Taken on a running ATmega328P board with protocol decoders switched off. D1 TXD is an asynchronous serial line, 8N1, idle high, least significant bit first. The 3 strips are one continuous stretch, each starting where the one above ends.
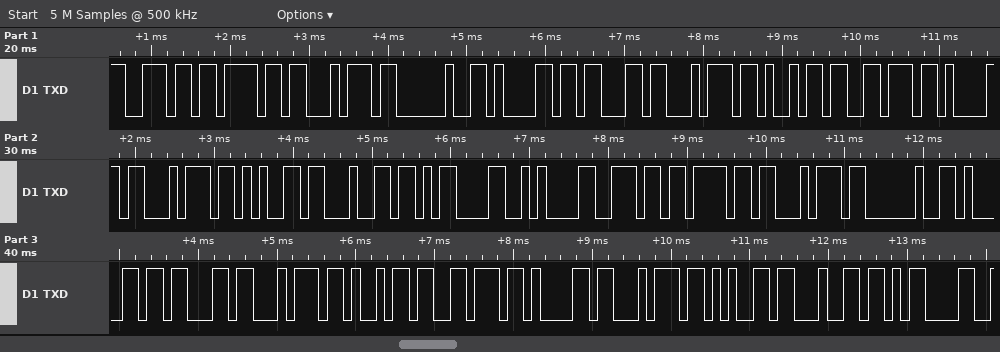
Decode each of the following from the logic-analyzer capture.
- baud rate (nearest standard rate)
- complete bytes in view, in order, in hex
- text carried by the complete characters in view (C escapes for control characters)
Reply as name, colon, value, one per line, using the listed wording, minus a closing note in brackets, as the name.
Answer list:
baud rate: 9600 baud
complete bytes in view, in order, in hex: 6E 6F 74 20 61 63 74 69 76 61 74 65 64 0D 0A 6E 6F 74 20 61 63 74 69 76 61 74 65 64 0D
text carried by the complete characters in view: "not activated\r\nnot activated\r"
